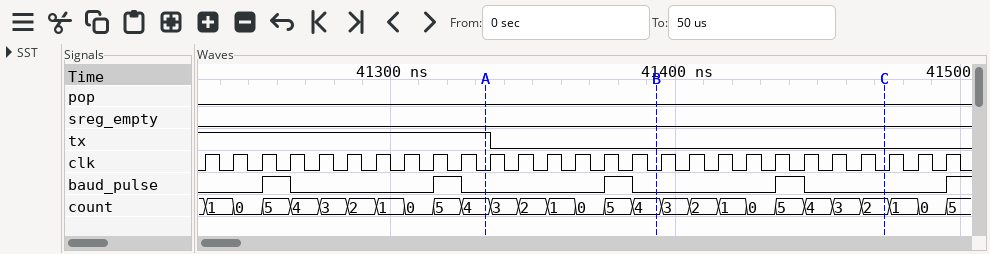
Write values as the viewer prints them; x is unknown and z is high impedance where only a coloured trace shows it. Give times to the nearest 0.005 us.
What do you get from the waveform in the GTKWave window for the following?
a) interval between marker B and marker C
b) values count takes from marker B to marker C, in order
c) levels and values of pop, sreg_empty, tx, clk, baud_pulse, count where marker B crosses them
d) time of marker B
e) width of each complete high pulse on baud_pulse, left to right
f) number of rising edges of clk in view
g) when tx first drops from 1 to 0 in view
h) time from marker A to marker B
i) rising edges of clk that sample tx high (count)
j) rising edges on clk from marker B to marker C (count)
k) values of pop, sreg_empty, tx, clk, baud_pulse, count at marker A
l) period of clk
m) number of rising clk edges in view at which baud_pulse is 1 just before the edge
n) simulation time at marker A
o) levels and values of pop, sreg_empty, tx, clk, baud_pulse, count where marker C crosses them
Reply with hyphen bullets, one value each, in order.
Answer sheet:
- 0.08 us
- 4, 3, 2, 1, 0, 5, 4, 3, 2
- pop=0, sreg_empty=0, tx=0, clk=0, baud_pulse=0, count=4
- 41.395 us
- 0.01 us, 0.01 us, 0.01 us, 0.01 us
- 27
- 41.335 us
- 0.06 us
- 11
- 8
- pop=0, sreg_empty=0, tx=1, clk=0, baud_pulse=0, count=4
- 0.01 us
- 4
- 41.335 us
- pop=0, sreg_empty=0, tx=0, clk=0, baud_pulse=0, count=2
